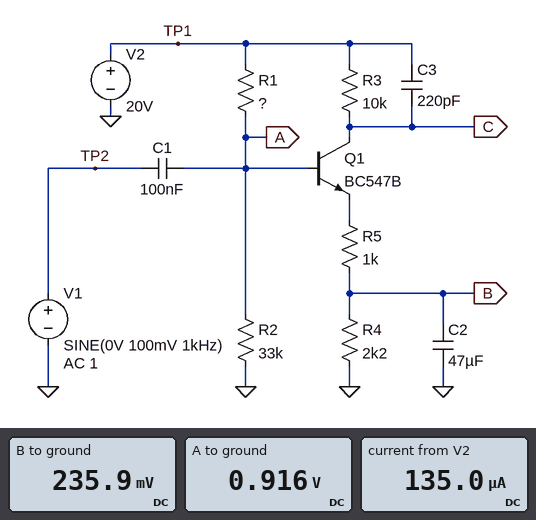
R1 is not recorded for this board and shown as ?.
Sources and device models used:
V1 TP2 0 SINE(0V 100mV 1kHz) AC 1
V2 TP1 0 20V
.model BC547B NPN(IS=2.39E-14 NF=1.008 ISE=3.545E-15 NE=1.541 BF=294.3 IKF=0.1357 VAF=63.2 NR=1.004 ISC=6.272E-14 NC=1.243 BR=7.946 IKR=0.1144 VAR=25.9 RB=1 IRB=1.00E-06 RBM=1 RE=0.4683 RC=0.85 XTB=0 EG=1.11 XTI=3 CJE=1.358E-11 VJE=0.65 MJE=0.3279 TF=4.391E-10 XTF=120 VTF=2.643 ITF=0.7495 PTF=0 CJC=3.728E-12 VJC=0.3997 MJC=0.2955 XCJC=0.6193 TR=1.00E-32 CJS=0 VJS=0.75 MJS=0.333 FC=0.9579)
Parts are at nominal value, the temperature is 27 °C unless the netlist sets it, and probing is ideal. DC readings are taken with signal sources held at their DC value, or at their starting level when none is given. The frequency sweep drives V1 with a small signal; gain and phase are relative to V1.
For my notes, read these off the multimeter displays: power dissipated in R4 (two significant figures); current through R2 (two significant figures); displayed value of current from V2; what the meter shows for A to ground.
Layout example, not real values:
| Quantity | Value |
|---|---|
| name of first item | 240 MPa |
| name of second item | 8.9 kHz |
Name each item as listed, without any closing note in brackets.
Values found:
| Quantity | Value |
|---|---|
| power dissipated in R4 | 25 µW |
| current through R2 | 28 µA |
| displayed value of current from V2 | 135.0 µA |
| what the meter shows for A to ground | 0.916 V |
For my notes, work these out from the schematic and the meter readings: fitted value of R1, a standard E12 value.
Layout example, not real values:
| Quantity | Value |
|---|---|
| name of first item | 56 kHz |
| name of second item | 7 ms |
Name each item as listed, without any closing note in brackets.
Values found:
| Quantity | Value |
|---|---|
| fitted value of R1, a standard E12 value | 680 kΩ |
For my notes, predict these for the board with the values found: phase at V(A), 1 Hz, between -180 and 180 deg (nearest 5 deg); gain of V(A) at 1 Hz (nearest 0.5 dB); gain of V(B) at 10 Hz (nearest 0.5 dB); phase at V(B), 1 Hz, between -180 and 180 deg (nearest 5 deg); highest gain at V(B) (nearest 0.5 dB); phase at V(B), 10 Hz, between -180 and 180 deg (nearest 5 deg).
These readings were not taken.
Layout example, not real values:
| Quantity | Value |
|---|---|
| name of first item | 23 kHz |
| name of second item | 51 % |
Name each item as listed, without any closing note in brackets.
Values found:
| Quantity | Value |
|---|---|
| phase at V(A), 1 Hz, between -180 and 180 deg | 90 deg |
| gain of V(A) at 1 Hz | -34.5 dB |
| gain of V(B) at 10 Hz | -27.0 dB |
| phase at V(B), 1 Hz, between -180 and 180 deg | 75 deg |
| highest gain at V(B) | -26.5 dB |
| phase at V(B), 10 Hz, between -180 and 180 deg | 10 deg |
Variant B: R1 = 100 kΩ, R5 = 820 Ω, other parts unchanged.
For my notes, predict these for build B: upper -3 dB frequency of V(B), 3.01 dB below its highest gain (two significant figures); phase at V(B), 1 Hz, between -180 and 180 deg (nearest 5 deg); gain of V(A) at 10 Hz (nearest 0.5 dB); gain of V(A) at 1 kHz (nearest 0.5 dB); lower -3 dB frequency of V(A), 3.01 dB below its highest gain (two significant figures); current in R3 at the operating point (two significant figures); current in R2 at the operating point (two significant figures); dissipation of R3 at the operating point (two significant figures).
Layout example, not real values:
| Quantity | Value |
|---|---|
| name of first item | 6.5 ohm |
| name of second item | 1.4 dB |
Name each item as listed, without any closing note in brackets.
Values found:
| Quantity | Value |
|---|---|
| upper -3 dB frequency of V(B), 3.01 dB below its highest gain | 82 Hz |
| phase at V(B), 1 Hz, between -180 and 180 deg | 80 deg |
| gain of V(A) at 10 Hz | -17.0 dB |
| gain of V(A) at 1 kHz | 0 dB |
| lower -3 dB frequency of V(A), 3.01 dB below its highest gain | 73 Hz |
| current in R3 at the operating point | 1.4 mA |
| current in R2 at the operating point | 150 µA |
| dissipation of R3 at the operating point | 19 mW |
